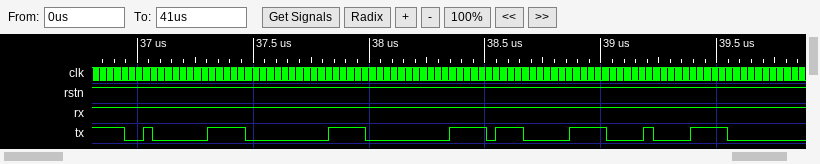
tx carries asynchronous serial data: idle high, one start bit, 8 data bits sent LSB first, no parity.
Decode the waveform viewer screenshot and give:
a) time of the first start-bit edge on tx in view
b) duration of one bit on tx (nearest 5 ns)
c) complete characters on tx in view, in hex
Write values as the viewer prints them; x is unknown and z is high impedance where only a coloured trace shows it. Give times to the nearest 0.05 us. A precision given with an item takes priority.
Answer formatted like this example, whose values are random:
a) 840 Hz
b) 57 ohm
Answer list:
a) 36.95 us
b) 40 ns
c) 02, 00, 00, 07, 08
